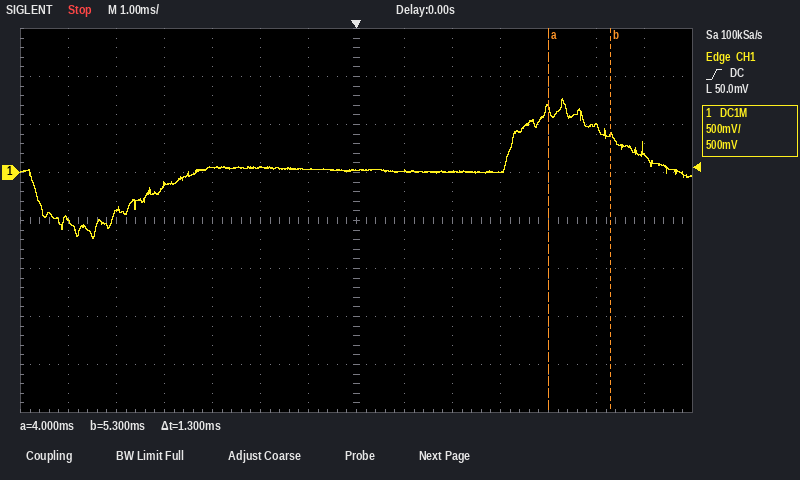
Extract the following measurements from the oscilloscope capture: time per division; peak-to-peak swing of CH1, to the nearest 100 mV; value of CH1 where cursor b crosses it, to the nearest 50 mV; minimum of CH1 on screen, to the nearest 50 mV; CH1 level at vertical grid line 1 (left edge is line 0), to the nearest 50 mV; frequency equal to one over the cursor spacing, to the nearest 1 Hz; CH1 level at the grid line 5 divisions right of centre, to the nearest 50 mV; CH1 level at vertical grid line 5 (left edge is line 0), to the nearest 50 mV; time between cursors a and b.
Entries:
1 ms
1.50 V
400 mV
-700 mV
-500 mV
769 Hz
500 mV
50 mV
1.3 ms
